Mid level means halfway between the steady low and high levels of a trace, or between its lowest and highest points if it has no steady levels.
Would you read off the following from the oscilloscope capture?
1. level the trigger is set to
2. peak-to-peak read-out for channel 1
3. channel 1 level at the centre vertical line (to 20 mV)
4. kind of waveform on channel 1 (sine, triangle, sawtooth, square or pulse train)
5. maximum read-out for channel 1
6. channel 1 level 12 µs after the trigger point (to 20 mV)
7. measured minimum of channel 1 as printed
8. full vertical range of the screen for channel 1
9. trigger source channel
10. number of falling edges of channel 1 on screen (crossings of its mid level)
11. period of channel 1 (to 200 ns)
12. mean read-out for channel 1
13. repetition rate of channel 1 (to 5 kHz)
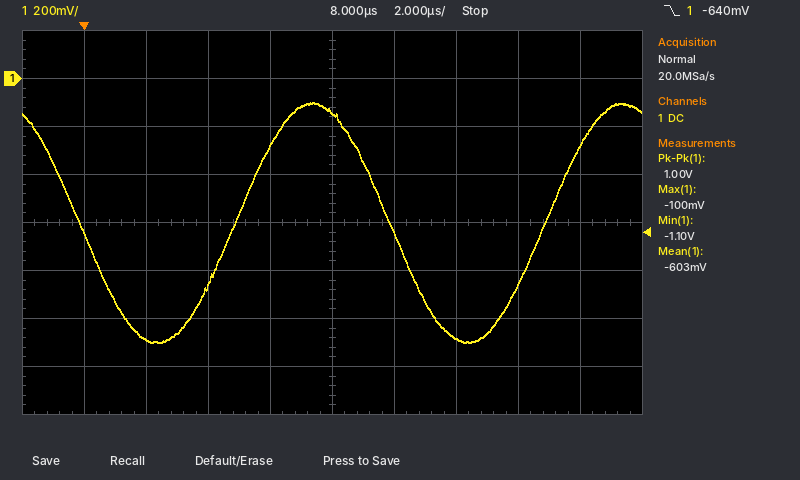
-640 mV
1.00 V
-140 mV
sine
-100 mV
-1.08 V
-1.10 V
1.6 V
channel 1
2
10.0 µs
-603 mV
100 kHz
